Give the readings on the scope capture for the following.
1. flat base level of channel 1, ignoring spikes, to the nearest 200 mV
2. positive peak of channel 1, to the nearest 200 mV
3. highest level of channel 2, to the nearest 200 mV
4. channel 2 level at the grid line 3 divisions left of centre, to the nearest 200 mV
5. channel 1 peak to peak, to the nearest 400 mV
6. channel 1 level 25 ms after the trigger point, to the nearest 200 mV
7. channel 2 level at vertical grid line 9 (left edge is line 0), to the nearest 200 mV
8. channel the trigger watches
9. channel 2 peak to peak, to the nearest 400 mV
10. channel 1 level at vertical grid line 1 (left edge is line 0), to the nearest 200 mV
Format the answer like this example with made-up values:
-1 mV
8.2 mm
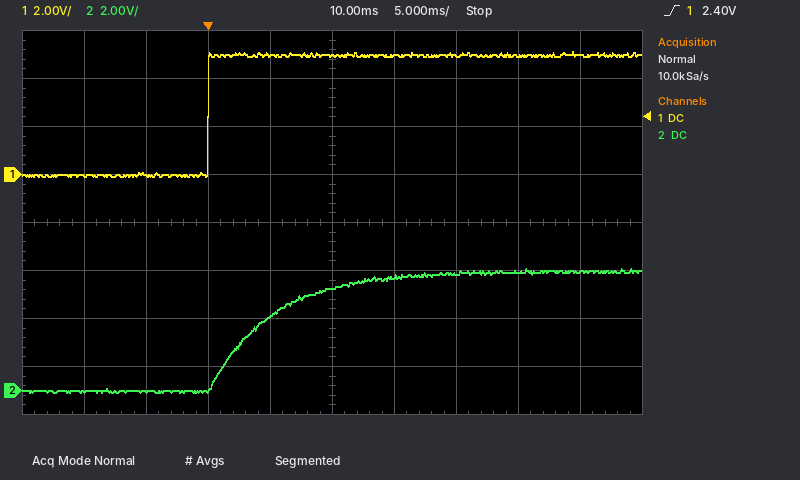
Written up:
0.0 V
5.2 V
5.0 V
0.0 V
5.2 V
5.0 V
5.0 V
channel 1
5.2 V
0.0 V
